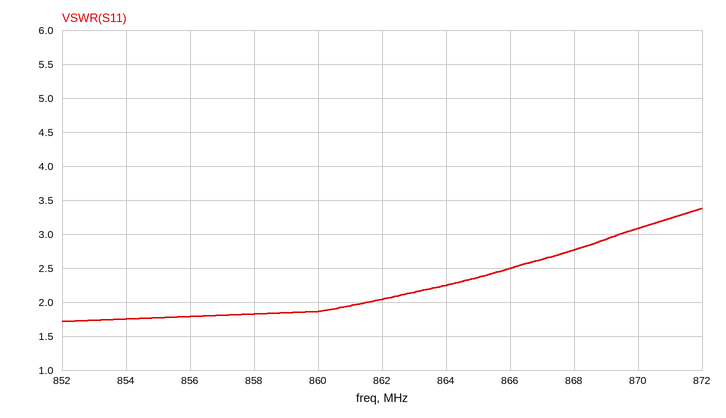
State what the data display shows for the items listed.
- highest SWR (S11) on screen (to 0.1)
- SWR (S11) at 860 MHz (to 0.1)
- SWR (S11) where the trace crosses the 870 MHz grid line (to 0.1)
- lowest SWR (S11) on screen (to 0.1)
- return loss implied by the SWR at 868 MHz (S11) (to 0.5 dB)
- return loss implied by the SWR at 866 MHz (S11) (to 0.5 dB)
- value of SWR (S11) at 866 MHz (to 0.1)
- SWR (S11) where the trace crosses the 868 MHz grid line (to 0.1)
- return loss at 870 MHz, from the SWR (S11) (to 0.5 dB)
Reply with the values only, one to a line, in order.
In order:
3.4
1.9
3.1
1.7
6.5 dB
7.5 dB
2.5
2.8
6.0 dB
